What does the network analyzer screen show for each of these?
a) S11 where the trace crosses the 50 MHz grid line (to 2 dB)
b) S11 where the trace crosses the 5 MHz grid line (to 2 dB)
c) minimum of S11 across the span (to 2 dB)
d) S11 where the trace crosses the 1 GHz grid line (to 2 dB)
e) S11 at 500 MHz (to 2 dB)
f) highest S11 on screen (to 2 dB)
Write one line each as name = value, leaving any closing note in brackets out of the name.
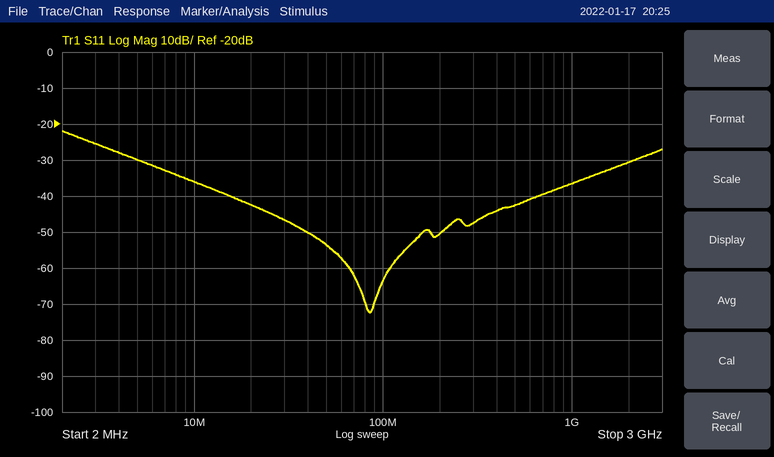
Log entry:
S11 where the trace crosses the 50 MHz grid line = -54 dB
S11 where the trace crosses the 5 MHz grid line = -30 dB
minimum of S11 across the span = -72 dB
S11 where the trace crosses the 1 GHz grid line = -36 dB
S11 at 500 MHz = -42 dB
highest S11 on screen = -22 dB
